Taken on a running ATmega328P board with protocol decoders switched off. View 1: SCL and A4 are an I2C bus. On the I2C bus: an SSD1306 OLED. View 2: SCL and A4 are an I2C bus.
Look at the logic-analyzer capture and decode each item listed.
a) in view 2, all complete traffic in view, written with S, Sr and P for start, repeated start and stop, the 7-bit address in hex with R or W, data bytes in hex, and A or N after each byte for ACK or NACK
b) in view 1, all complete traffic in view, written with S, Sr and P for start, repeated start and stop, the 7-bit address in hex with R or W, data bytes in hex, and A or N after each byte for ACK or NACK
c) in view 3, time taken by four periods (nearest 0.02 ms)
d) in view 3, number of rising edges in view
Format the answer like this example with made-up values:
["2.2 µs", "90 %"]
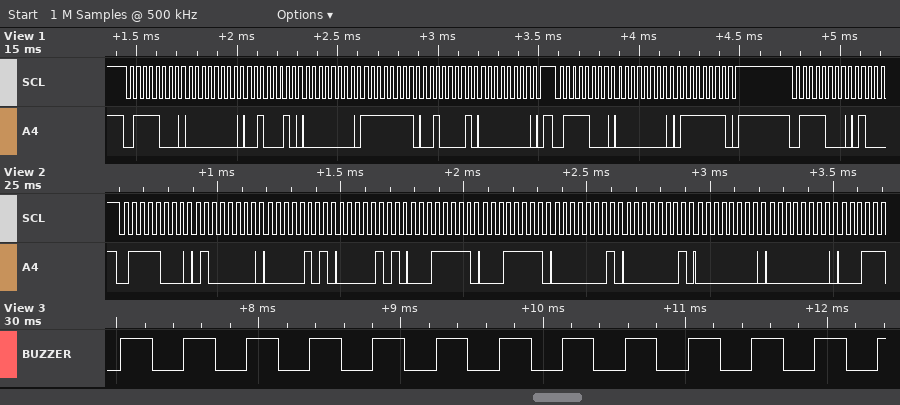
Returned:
["S 3CW A 40 A 05 A 05 A 1F A 1F A 01 A 01 A 00 A 00 A", "S 3CW A 00 A 22 A 00 A FF A 21 A 00 A P S 3CW A 00 A 7F A P S 3CW A", "1.78 ms", "13"]
